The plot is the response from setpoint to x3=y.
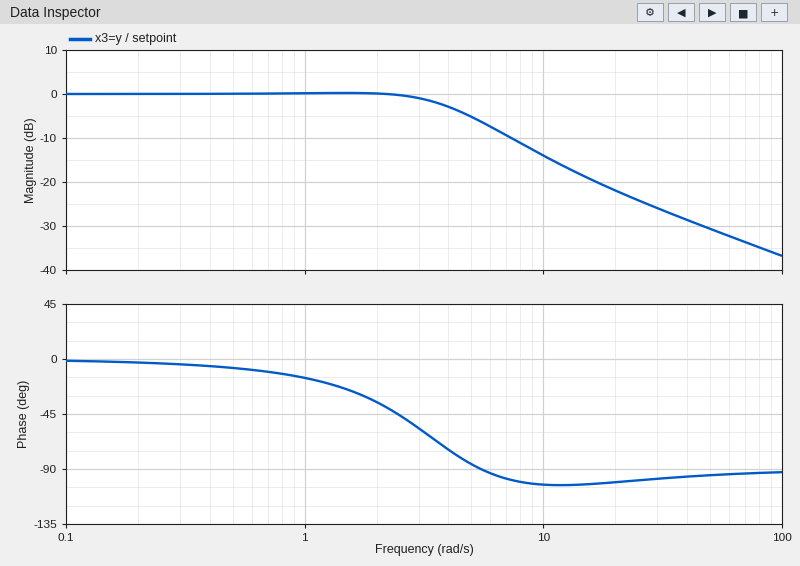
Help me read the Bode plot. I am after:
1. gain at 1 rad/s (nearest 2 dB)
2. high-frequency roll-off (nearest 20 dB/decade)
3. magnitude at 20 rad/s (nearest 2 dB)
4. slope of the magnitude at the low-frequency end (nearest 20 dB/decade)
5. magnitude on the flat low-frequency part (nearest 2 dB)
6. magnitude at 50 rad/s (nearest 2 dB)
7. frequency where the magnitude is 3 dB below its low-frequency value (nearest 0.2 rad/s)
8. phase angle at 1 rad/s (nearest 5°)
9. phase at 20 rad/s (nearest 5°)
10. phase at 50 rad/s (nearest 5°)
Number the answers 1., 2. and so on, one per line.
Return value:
1. 0 dB
2. -20 dB/decade
3. -22 dB
4. 0 dB/decade
5. 0 dB
6. -30 dB
7. 4.0 rad/s
8. -15°
9. -100°
10. -95°
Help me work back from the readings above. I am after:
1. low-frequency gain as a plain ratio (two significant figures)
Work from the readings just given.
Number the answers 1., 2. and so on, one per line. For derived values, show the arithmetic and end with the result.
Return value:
1. 10^(0 / 20) = 1.0
